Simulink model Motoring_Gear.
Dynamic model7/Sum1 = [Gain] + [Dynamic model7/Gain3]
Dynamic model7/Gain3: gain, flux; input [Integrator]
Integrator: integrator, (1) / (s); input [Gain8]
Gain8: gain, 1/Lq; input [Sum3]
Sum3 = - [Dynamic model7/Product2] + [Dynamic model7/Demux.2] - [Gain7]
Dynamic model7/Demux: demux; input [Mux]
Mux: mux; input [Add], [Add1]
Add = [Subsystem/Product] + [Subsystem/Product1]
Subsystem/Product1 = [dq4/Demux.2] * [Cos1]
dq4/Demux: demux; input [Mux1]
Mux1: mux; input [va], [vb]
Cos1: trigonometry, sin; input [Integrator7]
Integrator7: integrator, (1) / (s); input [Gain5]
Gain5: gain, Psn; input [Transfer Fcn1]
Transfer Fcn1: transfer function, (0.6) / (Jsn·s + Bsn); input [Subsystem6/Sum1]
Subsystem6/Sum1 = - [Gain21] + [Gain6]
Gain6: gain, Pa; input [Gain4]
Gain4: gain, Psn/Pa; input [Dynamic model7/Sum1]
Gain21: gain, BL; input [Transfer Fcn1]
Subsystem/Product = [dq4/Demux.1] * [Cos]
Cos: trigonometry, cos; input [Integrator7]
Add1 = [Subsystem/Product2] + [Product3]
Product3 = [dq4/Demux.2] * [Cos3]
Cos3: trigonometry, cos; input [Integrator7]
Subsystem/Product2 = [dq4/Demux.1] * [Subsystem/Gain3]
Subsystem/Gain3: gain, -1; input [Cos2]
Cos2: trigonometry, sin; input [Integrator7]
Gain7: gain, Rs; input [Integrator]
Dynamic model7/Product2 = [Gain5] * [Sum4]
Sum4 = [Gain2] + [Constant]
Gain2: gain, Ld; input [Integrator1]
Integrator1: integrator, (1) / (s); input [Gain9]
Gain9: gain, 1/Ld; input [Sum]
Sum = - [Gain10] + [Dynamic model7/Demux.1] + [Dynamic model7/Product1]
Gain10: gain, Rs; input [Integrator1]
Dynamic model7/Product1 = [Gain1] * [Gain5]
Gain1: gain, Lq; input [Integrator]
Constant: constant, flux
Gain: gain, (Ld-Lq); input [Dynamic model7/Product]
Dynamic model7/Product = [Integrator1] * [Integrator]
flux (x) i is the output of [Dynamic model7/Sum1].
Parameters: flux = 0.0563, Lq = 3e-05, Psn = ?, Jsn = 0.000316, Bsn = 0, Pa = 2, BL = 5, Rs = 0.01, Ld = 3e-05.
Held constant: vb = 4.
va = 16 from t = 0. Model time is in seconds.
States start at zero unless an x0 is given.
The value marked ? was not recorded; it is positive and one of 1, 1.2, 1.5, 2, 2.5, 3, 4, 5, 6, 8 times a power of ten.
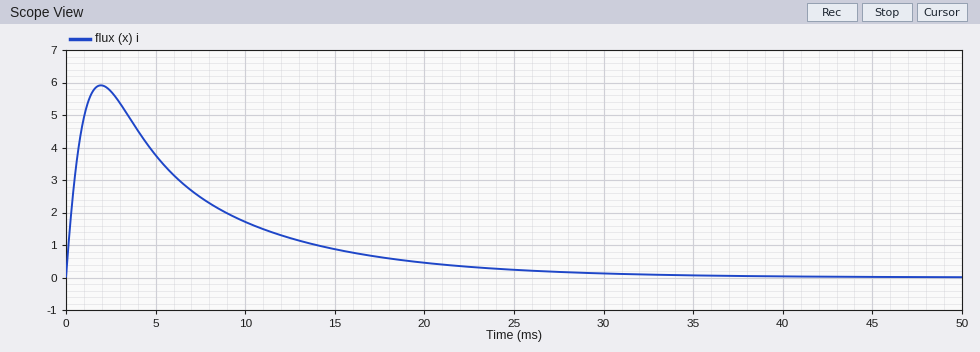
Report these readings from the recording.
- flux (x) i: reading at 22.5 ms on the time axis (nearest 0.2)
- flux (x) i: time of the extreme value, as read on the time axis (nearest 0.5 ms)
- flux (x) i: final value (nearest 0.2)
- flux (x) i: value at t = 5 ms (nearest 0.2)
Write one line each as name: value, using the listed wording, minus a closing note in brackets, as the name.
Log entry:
flux (x) i: reading at 22.5 ms on the time axis: 0.4
flux (x) i: time of the extreme value, as read on the time axis: 2.0 ms
flux (x) i: final value: 0.0
flux (x) i: value at t = 5 ms: 3.8
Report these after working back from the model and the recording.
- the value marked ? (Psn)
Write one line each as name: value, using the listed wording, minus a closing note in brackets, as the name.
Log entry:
the value marked ?: 5
